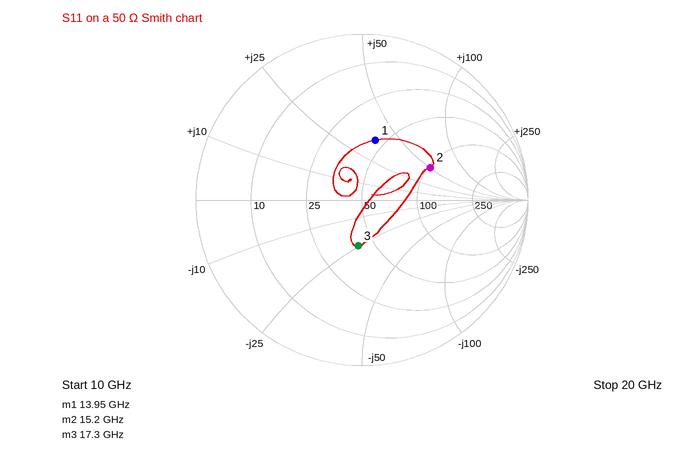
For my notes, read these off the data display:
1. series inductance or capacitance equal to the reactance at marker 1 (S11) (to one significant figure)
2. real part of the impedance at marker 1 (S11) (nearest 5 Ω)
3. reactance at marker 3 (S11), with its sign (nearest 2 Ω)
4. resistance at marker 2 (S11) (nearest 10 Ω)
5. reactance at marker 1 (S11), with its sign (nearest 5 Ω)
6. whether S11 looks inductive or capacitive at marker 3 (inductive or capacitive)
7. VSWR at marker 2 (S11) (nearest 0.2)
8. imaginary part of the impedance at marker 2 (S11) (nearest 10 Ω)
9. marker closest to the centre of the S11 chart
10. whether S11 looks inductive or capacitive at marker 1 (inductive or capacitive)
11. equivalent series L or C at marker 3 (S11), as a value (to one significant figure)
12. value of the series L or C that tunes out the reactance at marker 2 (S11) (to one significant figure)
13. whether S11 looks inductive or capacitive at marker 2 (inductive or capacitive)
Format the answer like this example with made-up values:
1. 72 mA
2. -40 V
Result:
1. 400 pH
2. 45 Ω
3. -24 Ω
4. 100 Ω
5. +35 Ω
6. capacitive
7. 2.6
8. +50 Ω
9. marker 3
10. inductive
11. 400 fF
12. 200 fF
13. inductive
